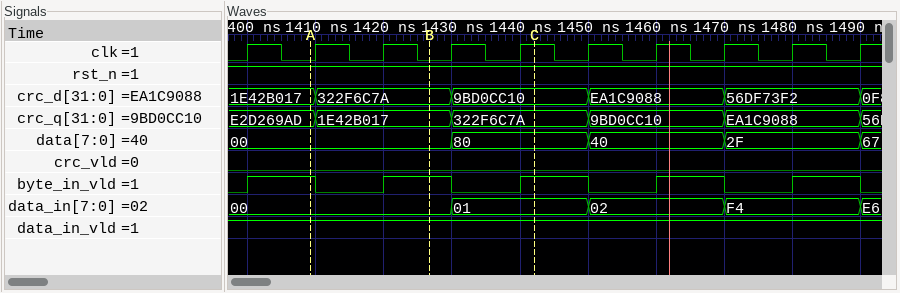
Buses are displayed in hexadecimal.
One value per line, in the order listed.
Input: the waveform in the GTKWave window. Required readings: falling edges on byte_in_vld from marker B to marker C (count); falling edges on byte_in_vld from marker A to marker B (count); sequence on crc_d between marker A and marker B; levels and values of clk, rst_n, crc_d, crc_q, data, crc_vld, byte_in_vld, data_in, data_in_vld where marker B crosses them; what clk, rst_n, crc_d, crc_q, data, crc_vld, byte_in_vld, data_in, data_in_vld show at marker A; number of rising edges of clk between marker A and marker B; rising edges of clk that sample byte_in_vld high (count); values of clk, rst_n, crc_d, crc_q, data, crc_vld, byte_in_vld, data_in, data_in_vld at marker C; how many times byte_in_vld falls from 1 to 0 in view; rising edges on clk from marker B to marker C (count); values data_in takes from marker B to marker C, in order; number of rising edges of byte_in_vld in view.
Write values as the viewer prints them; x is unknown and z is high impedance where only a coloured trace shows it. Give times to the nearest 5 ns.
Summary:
1
1
1E42B017, 322F6C7A
clk=0, rst_n=1, crc_d=322F6C7A, crc_q=1E42B017, data=00, crc_vld=0, byte_in_vld=1, data_in=00, data_in_vld=1
clk=0, rst_n=1, crc_d=1E42B017, crc_q=E2D269AD, data=00, crc_vld=0, byte_in_vld=1, data_in=00, data_in_vld=1
2
5
clk=1, rst_n=1, crc_d=9BD0CC10, crc_q=322F6C7A, data=80, crc_vld=0, byte_in_vld=1, data_in=01, data_in_vld=1
5
2
00, 01
5
